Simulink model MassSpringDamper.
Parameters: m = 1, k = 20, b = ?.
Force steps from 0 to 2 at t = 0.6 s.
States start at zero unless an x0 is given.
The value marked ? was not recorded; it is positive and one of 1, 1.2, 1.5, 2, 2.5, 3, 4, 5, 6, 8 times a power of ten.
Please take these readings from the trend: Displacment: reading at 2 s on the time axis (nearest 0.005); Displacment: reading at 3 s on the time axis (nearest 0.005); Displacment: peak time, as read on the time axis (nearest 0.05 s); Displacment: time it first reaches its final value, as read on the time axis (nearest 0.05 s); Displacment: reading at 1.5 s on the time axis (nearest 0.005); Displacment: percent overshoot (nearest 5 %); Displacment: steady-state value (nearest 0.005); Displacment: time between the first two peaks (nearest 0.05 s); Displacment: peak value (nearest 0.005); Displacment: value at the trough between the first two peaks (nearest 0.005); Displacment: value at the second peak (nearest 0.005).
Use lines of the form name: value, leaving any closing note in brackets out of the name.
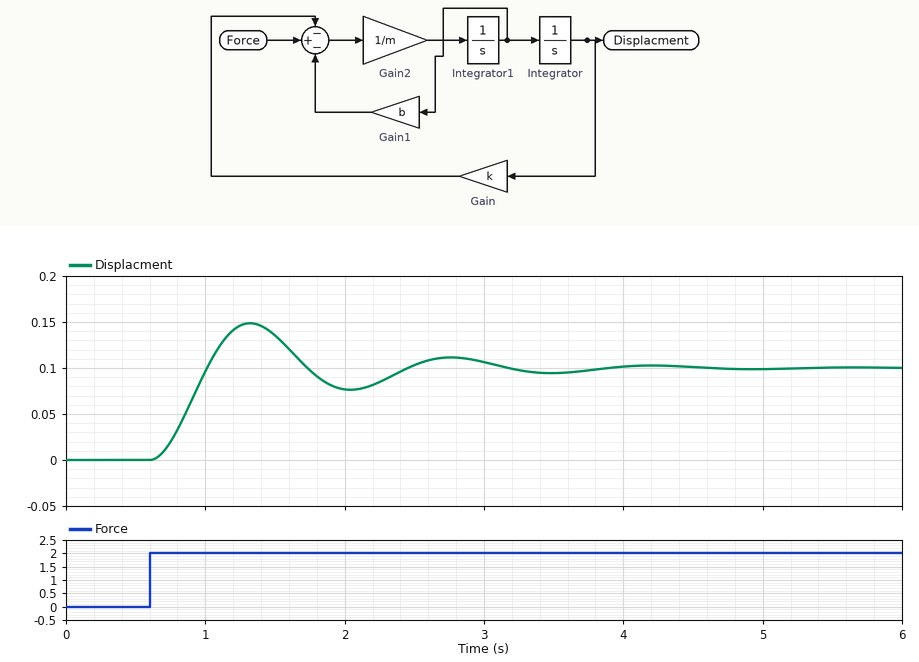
Displacment: reading at 2 s on the time axis: 0.075
Displacment: reading at 3 s on the time axis: 0.105
Displacment: peak time, as read on the time axis: 1.30 s
Displacment: time it first reaches its final value, as read on the time axis: 1.00 s
Displacment: reading at 1.5 s on the time axis: 0.135
Displacment: percent overshoot: 50 %
Displacment: steady-state value: 0.100
Displacment: time between the first two peaks: 1.45 s
Displacment: peak value: 0.150
Displacment: value at the trough between the first two peaks: 0.075
Displacment: value at the second peak: 0.110
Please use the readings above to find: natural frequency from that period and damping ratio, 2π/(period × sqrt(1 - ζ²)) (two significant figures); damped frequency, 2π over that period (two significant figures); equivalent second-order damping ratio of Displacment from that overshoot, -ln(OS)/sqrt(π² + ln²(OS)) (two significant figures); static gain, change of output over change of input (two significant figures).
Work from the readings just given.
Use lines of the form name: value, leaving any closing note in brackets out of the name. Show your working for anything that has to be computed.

natural frequency from that period and damping ratio, 2π/(period × sqrt(1 - ζ²)): 2π / (1.45 × sqrt(1 - 0.22²)) = 4.4 rad/s
damped frequency, 2π over that period: 2π / 1.45 = 4.3 rad/s
equivalent second-order damping ratio of Displacment from that overshoot, -ln(OS)/sqrt(π² + ln²(OS)): ln(0.5) = -0.693; 0.693 / sqrt(9.870 + 0.480) = 0.22
static gain, change of output over change of input: (0.1 - 0) / (2 - 0) = 0.050
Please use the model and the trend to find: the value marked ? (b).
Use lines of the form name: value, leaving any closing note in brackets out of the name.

the value marked ?: 2
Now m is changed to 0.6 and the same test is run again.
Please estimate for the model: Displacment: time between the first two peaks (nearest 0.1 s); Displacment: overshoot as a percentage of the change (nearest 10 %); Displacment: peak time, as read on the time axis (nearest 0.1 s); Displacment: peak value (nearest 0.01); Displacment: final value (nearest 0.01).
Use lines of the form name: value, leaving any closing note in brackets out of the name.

Displacment: time between the first two peaks: 1.1 s
Displacment: overshoot as a percentage of the change: 40 %
Displacment: peak time, as read on the time axis: 1.2 s
Displacment: peak value: 0.14
Displacment: final value: 0.10
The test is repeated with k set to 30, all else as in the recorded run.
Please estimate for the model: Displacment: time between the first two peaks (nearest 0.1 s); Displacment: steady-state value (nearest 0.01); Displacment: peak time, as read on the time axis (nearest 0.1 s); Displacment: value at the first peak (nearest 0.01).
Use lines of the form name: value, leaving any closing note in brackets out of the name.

Displacment: time between the first two peaks: 1.2 s
Displacment: steady-state value: 0.07
Displacment: peak time, as read on the time axis: 1.2 s
Displacment: value at the first peak: 0.10
